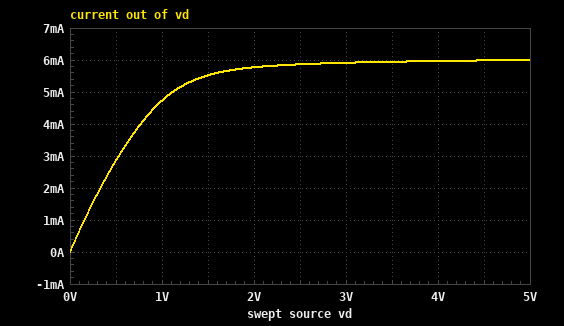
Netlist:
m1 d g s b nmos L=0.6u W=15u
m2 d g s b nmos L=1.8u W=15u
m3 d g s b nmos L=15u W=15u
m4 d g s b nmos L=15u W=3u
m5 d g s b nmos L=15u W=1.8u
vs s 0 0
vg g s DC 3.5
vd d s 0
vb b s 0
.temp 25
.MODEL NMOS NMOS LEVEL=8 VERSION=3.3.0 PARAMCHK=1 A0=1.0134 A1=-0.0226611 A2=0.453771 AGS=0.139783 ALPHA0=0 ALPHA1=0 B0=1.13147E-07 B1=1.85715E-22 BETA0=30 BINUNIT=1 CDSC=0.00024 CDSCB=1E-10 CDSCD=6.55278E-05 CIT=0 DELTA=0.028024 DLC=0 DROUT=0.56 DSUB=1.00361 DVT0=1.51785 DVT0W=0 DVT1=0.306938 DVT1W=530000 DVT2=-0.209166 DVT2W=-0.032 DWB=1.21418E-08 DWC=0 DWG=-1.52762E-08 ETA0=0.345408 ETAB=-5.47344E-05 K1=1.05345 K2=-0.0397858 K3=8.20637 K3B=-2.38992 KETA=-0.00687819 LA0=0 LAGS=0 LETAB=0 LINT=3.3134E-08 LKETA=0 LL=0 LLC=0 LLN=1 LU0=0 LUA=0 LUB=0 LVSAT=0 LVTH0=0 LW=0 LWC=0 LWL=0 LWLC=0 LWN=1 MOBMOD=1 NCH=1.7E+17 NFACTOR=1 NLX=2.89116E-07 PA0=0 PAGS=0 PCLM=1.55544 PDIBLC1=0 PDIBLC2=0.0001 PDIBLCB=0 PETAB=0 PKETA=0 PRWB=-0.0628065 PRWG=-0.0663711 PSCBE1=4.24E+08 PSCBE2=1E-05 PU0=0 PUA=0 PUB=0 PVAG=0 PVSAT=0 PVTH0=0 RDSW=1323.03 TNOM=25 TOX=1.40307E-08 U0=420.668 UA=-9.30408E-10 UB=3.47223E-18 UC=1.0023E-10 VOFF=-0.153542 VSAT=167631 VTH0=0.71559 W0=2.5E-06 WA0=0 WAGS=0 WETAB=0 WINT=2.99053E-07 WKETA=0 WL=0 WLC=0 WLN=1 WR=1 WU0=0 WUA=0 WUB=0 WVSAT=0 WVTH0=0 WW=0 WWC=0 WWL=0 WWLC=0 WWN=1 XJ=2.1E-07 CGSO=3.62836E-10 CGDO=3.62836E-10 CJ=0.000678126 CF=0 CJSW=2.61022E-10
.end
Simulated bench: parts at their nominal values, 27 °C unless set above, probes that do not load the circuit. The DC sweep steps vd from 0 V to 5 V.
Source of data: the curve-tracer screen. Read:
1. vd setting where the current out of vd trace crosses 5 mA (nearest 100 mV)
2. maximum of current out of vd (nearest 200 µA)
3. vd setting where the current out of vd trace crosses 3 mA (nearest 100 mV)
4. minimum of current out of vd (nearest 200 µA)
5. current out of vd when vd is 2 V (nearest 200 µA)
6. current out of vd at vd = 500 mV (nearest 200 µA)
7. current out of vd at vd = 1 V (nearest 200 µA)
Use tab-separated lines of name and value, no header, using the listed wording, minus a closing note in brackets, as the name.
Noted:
vd setting where the current out of vd trace crosses 5 mA	1.1 V
maximum of current out of vd	6.0 mA
vd setting where the current out of vd trace crosses 3 mA	500 mV
minimum of current out of vd	0 A
current out of vd when vd is 2 V	5.8 mA
current out of vd at vd = 500 mV	2.8 mA
current out of vd at vd = 1 V	4.8 mA
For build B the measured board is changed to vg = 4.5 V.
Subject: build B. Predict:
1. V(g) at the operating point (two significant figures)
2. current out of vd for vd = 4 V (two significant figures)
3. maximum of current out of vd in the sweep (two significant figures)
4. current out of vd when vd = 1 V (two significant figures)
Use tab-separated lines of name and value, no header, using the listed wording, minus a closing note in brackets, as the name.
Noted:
V(g) at the operating point	4.5 V
current out of vd for vd = 4 V	9.1 mA
maximum of current out of vd in the sweep	9.2 mA
current out of vd when vd = 1 V	6.3 mA
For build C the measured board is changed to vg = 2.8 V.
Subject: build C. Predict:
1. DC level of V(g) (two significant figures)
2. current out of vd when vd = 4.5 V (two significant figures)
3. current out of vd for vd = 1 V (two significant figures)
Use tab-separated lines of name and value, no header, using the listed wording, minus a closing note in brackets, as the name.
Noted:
DC level of V(g)	2.8 V
current out of vd when vd = 4.5 V	3.9 mA
current out of vd for vd = 1 V	3.3 mA
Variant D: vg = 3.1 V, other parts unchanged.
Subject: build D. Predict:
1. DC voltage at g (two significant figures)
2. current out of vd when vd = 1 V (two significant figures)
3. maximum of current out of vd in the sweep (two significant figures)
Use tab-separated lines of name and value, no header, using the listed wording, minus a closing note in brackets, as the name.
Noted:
DC voltage at g	3.1 V
current out of vd when vd = 1 V	4.0 mA
maximum of current out of vd in the sweep	4.8 mA
